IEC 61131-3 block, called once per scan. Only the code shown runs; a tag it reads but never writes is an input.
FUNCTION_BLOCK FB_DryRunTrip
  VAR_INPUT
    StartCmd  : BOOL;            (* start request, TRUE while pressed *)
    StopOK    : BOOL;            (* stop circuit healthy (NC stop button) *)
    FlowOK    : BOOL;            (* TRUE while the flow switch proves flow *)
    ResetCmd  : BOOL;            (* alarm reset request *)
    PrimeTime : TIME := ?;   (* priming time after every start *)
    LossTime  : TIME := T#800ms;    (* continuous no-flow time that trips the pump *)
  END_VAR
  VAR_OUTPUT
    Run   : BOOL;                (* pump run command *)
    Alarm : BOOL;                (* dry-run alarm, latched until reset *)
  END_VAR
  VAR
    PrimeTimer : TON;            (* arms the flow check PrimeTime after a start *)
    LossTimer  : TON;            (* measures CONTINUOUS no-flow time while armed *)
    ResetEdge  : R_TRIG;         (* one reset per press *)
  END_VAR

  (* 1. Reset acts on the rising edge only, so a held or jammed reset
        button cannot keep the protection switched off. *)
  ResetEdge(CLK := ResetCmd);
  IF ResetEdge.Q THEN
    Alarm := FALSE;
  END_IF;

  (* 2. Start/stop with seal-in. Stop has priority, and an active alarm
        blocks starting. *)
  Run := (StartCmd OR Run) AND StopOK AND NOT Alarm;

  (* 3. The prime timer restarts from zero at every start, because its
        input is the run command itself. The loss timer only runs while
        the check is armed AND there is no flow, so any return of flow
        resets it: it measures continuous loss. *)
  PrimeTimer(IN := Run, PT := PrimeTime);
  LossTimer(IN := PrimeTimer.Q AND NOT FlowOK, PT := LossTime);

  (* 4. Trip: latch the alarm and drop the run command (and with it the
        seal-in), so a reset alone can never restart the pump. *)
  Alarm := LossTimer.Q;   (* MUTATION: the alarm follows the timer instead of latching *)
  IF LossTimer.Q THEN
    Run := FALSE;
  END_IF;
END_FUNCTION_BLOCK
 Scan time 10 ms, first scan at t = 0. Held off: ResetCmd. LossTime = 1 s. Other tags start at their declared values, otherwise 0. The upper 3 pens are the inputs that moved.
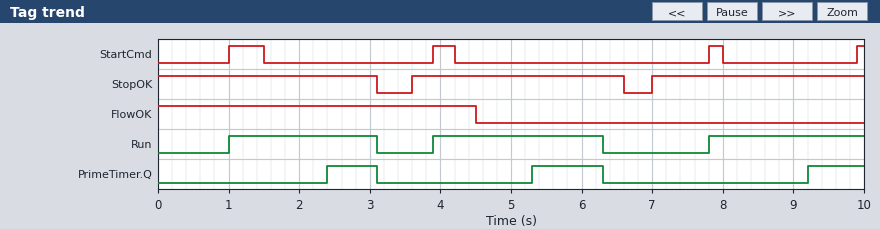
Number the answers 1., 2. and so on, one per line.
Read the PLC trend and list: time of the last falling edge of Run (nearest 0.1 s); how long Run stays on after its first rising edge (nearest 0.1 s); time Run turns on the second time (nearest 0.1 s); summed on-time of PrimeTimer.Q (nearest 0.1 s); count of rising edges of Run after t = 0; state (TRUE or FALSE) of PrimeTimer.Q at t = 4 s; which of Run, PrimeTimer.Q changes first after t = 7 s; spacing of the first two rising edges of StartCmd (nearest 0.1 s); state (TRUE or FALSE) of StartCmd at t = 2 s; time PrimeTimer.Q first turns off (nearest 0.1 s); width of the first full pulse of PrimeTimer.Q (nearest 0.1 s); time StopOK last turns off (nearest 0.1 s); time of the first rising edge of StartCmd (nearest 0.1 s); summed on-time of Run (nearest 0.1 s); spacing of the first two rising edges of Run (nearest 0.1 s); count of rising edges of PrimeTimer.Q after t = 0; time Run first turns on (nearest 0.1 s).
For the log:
1. 6.3 s
2. 2.1 s
3. 3.9 s
4. 2.5 s
5. 3
6. FALSE
7. Run
8. 2.9 s
9. FALSE
10. 3.1 s
11. 0.7 s
12. 6.6 s
13. 1.0 s
14. 6.7 s
15. 2.9 s
16. 3
17. 1.0 s
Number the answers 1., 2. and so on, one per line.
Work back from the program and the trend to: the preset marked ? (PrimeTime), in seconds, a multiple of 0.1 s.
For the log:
1. 1.4 s
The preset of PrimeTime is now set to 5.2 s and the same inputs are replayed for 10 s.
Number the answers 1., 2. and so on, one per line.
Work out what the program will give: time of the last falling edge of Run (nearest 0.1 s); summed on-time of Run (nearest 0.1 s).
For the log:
1. 6.6 s
2. 7.0 s
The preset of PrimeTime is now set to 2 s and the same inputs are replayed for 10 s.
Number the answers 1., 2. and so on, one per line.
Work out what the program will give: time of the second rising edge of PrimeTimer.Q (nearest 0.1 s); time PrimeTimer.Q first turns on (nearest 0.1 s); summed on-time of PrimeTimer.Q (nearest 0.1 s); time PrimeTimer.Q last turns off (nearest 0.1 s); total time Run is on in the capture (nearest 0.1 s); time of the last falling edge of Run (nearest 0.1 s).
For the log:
1. 5.9 s
2. 3.0 s
3. 1.0 s
4. 6.6 s
5. 7.0 s
6. 6.6 s
